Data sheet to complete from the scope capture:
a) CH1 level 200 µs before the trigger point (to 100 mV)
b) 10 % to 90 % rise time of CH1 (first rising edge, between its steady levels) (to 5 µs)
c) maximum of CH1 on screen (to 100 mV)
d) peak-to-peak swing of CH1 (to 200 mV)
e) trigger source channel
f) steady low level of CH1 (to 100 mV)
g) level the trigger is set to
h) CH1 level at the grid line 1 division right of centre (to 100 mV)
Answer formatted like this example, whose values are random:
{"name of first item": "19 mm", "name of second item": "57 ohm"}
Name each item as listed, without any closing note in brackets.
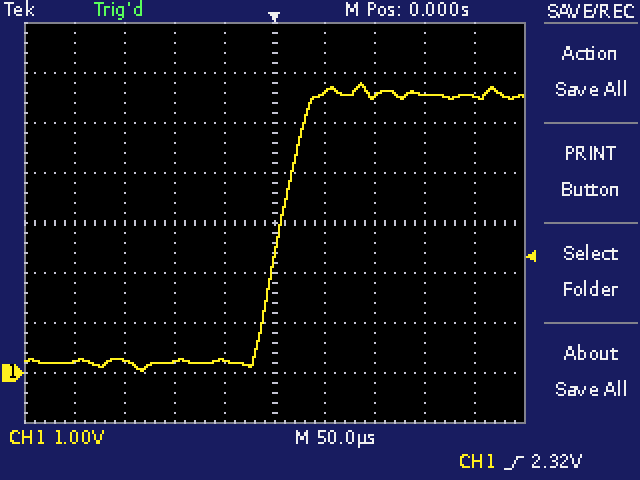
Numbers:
{"CH1 level 200 µs before the trigger point": "200 mV", "10 % to 90 % rise time of CH1 (first rising edge, between its steady levels)": "45 µs", "maximum of CH1 on screen": "5.8 V", "peak-to-peak swing of CH1": "5.8 V", "trigger source channel": "CH1", "steady low level of CH1": "200 mV", "level the trigger is set to": "2.32 V", "CH1 level at the grid line 1 division right of centre": "5.6 V"}
